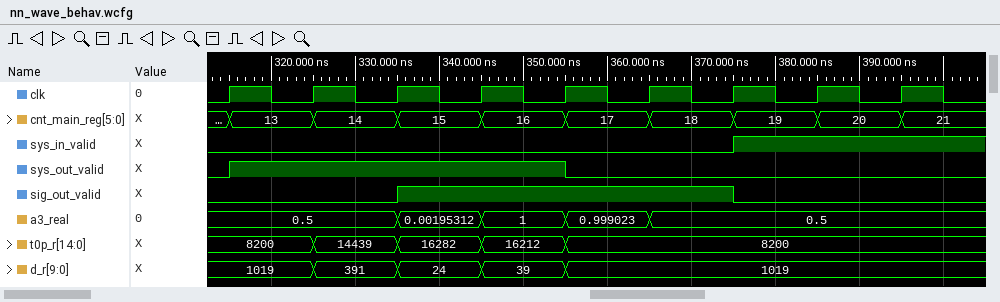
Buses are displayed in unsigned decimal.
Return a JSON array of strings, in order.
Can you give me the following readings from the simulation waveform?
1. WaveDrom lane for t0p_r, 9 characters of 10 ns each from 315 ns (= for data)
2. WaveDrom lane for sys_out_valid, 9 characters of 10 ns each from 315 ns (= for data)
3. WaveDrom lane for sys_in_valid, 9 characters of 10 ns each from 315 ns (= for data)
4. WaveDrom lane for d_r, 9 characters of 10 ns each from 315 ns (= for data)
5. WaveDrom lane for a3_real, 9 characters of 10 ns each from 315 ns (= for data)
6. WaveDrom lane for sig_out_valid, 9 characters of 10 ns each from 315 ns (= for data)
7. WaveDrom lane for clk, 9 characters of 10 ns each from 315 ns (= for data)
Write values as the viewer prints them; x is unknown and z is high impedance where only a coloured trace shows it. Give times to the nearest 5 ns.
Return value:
["{name: 't0p_r', wave: '=====....', data: '8200 14439 16282 16212 8200'}", "{name: 'sys_out_valid', wave: '1...0....'}", "{name: 'sys_in_valid', wave: '0.....1..'}", "{name: 'd_r', wave: '=====....', data: '1019 391 24 39 1019'}", "{name: 'a3_real', wave: '=.====...', data: '0.5 0.00195312 1 0.999023 0.5'}", "{name: 'sig_out_valid', wave: '0.1...0..'}", "{name: 'clk', wave: 'p........'}"]
